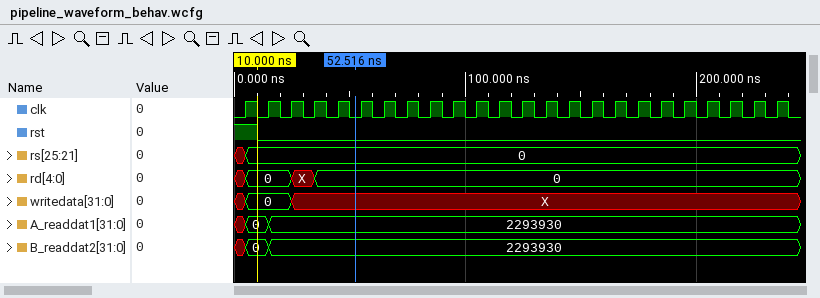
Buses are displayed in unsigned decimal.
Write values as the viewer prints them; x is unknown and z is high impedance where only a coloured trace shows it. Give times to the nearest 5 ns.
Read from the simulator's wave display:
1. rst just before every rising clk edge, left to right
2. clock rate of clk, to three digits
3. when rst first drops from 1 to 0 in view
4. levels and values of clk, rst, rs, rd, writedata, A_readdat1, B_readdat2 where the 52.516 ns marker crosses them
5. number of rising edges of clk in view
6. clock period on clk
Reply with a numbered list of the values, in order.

1. 1 0 0 0 0 0 0 0 0 0 0 0 0 0 0 0 0 0 0 0 0 0 0 0
2. 100 MHz
3. 10 ns
4. clk=0, rst=0, rs=0, rd=0, writedata=X, A_readdat1=2293930, B_readdat2=2293930
5. 24
6. 10 ns
